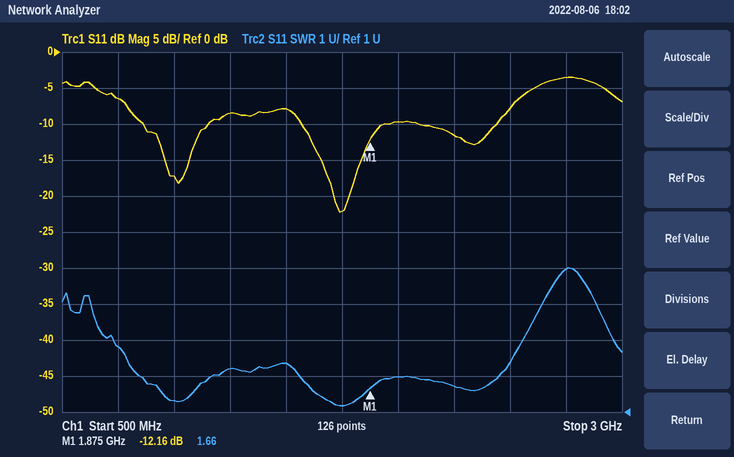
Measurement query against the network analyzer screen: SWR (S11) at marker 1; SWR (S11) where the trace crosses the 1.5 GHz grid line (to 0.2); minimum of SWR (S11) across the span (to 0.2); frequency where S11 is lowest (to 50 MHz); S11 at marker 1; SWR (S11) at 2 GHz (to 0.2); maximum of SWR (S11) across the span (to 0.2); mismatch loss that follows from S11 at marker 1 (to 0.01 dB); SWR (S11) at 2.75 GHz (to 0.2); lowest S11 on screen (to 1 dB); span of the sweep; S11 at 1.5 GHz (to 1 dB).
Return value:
1.66
2.4
1.2
1.75 GHz
-12.16 dB
2.0
5.0
0.27 dB
5.0
-22 dB
2.5 GHz
-8 dB
